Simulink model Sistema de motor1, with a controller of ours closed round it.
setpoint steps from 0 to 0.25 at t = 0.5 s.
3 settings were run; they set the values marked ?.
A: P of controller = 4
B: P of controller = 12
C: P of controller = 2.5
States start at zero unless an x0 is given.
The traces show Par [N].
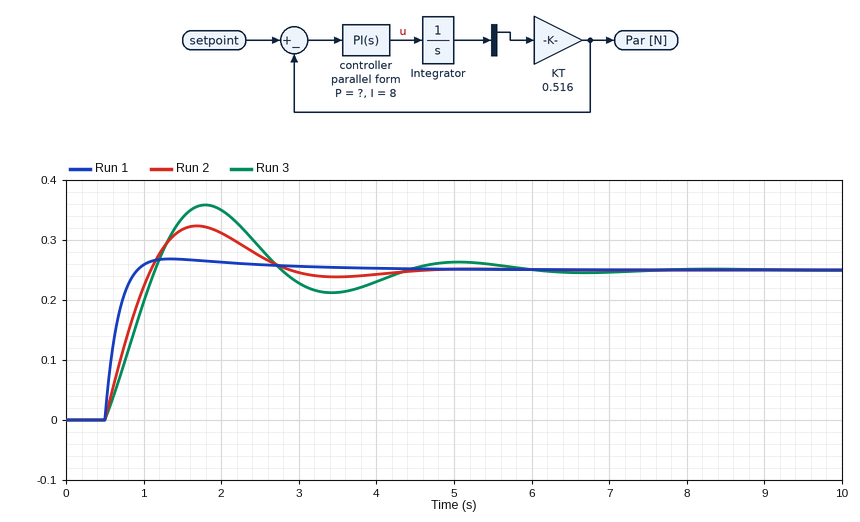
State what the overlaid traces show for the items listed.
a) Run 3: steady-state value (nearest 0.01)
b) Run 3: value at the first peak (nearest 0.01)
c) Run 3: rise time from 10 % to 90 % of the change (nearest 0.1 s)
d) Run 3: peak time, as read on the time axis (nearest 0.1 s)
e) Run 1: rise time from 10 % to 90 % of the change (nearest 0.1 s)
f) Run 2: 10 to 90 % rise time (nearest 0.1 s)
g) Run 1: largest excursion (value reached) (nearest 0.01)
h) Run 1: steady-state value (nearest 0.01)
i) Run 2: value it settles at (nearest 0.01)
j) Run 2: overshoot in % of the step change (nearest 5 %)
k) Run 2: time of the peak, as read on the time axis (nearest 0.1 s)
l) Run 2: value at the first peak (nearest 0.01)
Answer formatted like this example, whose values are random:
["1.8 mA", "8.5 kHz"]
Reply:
["0.25", "0.36", "0.5 s", "1.8 s", "0.3 s", "0.5 s", "0.27", "0.25", "0.25", "30 %", "1.7 s", "0.32"]
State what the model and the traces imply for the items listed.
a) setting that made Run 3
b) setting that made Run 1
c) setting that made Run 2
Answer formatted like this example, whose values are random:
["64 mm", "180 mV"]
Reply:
["C", "B", "A"]
